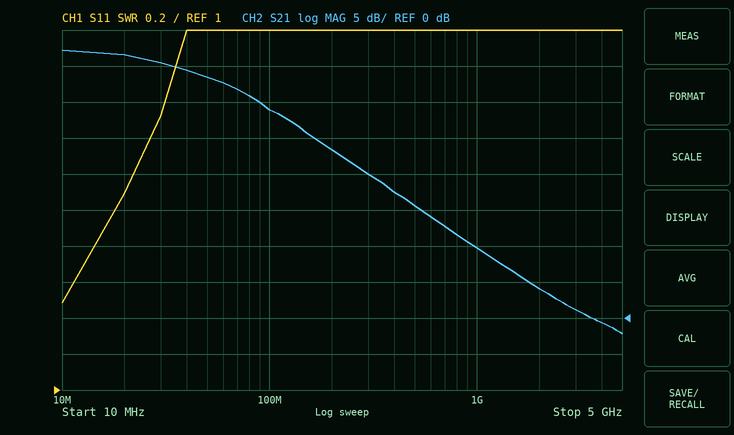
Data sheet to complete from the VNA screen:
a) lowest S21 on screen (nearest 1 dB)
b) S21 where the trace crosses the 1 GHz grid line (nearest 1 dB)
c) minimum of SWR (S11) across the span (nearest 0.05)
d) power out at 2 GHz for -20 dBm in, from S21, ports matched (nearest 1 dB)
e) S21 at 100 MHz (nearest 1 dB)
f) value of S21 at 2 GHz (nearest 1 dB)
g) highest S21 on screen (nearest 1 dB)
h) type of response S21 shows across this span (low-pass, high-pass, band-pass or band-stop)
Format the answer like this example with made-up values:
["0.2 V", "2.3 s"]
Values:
["-2 dB", "10 dB", "1.50", "-16 dBm", "29 dB", "4 dB", "37 dB", "low-pass"]
